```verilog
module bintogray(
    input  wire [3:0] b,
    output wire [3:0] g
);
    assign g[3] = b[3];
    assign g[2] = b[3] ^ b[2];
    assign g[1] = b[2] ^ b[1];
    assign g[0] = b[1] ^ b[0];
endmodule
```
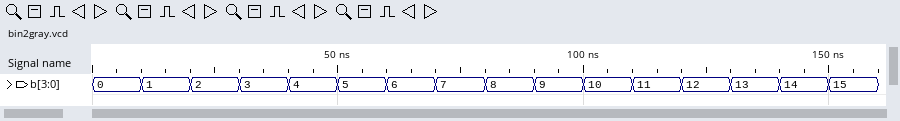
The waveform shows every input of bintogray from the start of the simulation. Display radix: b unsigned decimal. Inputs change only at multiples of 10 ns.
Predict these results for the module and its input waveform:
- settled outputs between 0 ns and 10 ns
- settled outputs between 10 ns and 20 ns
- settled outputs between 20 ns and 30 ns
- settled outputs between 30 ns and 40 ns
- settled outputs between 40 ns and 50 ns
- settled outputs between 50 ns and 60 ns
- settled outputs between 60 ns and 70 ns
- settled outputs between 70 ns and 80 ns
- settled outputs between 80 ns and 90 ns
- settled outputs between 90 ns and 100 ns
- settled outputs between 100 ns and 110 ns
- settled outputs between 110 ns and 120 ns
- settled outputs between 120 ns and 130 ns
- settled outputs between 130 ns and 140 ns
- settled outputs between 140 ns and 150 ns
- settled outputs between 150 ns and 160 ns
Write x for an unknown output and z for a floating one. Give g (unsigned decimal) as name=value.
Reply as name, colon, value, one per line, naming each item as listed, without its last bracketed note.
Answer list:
settled outputs between 0 ns and 10 ns: g=0
settled outputs between 10 ns and 20 ns: g=1
settled outputs between 20 ns and 30 ns: g=3
settled outputs between 30 ns and 40 ns: g=2
settled outputs between 40 ns and 50 ns: g=6
settled outputs between 50 ns and 60 ns: g=7
settled outputs between 60 ns and 70 ns: g=5
settled outputs between 70 ns and 80 ns: g=4
settled outputs between 80 ns and 90 ns: g=12
settled outputs between 90 ns and 100 ns: g=13
settled outputs between 100 ns and 110 ns: g=15
settled outputs between 110 ns and 120 ns: g=14
settled outputs between 120 ns and 130 ns: g=10
settled outputs between 130 ns and 140 ns: g=11
settled outputs between 140 ns and 150 ns: g=9
settled outputs between 150 ns and 160 ns: g=8
